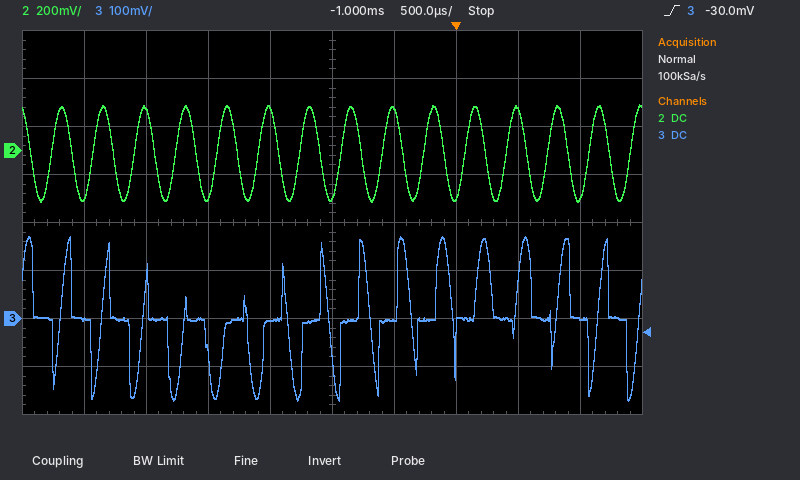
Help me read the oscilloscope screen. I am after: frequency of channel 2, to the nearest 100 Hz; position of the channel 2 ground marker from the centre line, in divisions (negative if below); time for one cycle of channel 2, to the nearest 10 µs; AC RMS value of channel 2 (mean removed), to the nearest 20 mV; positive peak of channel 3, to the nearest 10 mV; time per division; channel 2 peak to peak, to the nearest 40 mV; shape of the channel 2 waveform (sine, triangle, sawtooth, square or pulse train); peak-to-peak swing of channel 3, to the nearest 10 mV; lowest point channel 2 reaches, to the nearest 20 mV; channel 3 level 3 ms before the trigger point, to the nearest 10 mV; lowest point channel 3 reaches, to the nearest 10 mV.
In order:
3.0 kHz
+1.5 div
330 µs
140 mV
170 mV
500 µs
400 mV
sine
340 mV
-220 mV
0 mV
-170 mV
